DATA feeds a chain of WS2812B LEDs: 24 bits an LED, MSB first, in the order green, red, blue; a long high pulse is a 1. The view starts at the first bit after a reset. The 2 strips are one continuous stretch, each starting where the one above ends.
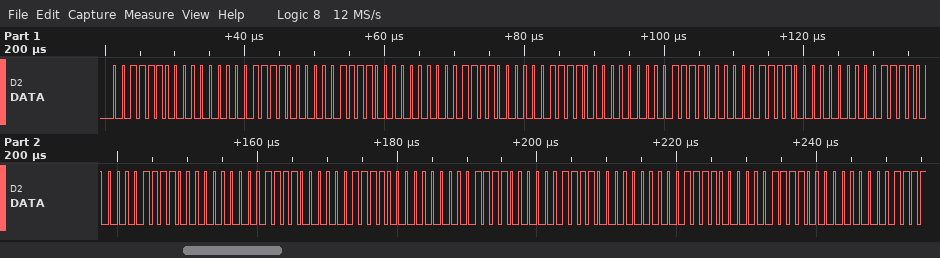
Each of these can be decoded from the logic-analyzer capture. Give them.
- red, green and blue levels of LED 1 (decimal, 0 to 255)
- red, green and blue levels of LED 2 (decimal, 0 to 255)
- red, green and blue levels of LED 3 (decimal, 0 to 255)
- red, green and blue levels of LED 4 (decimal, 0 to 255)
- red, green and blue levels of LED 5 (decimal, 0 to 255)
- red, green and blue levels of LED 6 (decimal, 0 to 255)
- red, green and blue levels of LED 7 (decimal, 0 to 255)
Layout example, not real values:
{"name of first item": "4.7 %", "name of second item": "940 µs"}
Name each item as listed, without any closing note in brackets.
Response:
{"red, green and blue levels of LED 1": "0, 60, 240", "red, green and blue levels of LED 2": "0, 60, 240", "red, green and blue levels of LED 3": "0, 60, 240", "red, green and blue levels of LED 4": "0, 60, 240", "red, green and blue levels of LED 5": "0, 60, 240", "red, green and blue levels of LED 6": "0, 60, 240", "red, green and blue levels of LED 7": "0, 60, 240"}
